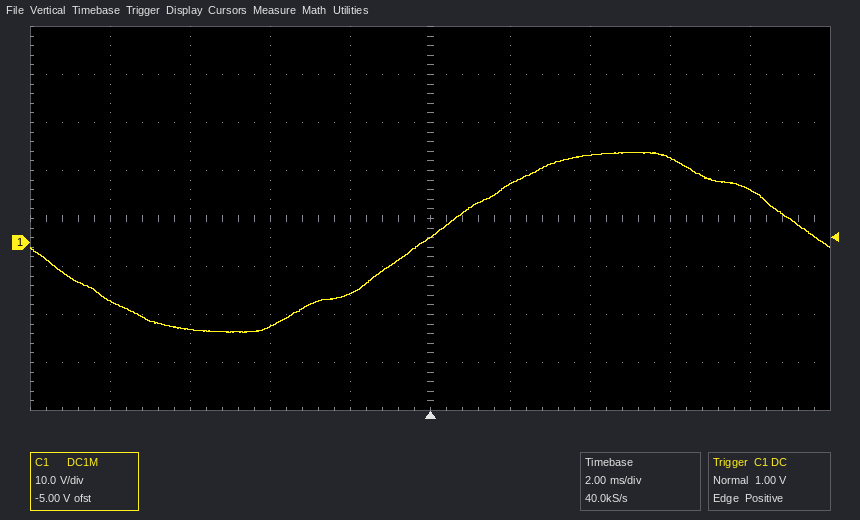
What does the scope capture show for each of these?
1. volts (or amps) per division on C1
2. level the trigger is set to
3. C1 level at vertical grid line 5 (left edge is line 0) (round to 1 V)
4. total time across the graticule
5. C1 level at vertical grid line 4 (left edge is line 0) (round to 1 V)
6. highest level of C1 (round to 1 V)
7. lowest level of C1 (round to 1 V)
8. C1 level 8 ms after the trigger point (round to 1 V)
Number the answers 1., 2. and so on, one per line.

1. 10 V
2. 1.00 V
3. 1 V
4. 20 ms
5. -11 V
6. 19 V
7. -19 V
8. 11 V
